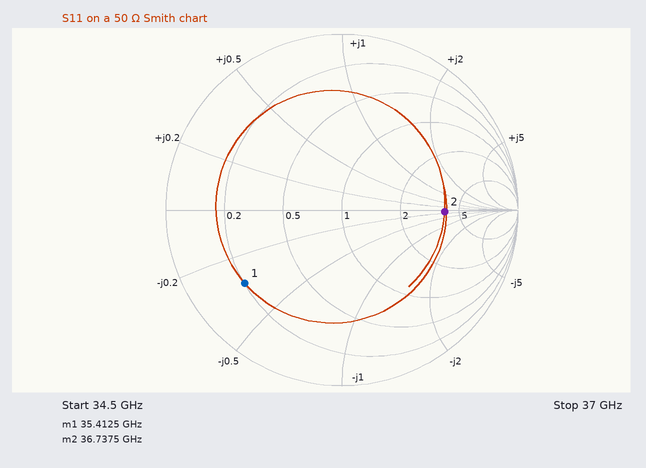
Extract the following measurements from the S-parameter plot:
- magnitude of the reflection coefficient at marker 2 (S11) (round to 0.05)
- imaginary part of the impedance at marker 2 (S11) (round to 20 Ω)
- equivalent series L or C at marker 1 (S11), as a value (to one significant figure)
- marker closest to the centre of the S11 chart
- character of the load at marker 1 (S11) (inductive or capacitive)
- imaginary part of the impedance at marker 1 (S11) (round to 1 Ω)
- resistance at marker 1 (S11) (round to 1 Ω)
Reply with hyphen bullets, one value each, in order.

- 0.60
- 0 Ω
- 300 fF
- marker 2
- capacitive
- -16 Ω
- 10 Ω
